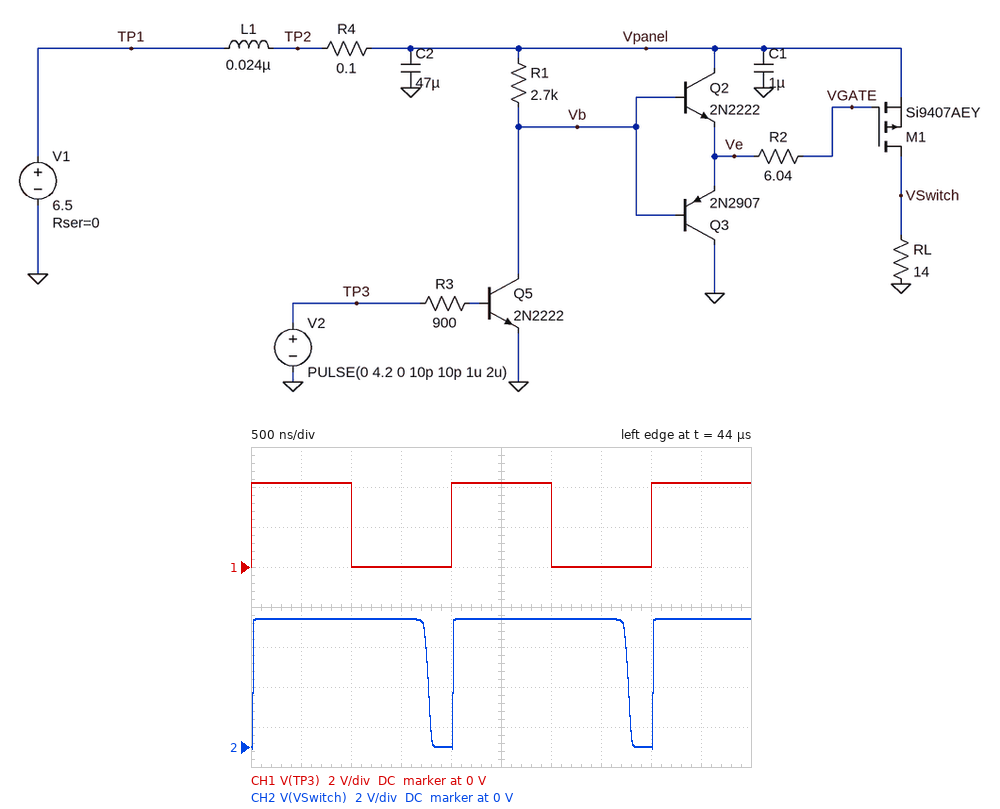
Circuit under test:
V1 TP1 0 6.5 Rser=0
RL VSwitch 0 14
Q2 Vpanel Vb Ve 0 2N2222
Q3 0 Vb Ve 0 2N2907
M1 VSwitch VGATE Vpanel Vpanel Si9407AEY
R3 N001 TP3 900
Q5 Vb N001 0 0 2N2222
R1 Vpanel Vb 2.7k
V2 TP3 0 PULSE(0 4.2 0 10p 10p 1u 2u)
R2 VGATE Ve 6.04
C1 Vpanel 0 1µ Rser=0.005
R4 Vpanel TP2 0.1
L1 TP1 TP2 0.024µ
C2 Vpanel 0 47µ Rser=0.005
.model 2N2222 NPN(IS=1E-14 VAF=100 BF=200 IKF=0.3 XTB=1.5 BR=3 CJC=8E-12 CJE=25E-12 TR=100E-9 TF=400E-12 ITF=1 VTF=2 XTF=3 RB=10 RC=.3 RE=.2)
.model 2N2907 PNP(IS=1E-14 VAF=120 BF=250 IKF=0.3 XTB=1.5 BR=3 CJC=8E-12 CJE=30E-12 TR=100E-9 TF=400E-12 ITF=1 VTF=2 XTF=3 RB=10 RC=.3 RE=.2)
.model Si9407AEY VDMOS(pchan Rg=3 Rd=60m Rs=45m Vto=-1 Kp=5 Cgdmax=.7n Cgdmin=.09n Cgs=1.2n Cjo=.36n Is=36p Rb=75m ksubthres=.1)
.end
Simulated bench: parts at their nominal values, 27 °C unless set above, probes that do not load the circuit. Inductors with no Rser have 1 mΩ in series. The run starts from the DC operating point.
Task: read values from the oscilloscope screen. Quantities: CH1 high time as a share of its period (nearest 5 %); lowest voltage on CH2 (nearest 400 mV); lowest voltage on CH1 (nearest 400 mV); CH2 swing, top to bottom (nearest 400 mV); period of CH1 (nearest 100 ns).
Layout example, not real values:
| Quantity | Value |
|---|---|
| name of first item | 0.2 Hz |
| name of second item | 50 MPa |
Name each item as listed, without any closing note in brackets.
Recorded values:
| Quantity | Value |
|---|---|
| CH1 high time as a share of its period | 50 % |
| lowest voltage on CH2 | 0 V |
| lowest voltage on CH1 | 0 V |
| CH2 swing, top to bottom | 6.4 V |
| period of CH1 | 2.0 µs |
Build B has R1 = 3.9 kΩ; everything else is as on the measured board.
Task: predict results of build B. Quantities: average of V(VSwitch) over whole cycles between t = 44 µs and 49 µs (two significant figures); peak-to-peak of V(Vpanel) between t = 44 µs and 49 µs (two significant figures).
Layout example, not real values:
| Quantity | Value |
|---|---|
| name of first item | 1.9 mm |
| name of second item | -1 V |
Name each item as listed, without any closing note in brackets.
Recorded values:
| Quantity | Value |
|---|---|
| average of V(VSwitch) over whole cycles between t = 44 µs and 49 µs | 5.9 V |
| peak-to-peak of V(Vpanel) between t = 44 µs and 49 µs | 3.3 mV |
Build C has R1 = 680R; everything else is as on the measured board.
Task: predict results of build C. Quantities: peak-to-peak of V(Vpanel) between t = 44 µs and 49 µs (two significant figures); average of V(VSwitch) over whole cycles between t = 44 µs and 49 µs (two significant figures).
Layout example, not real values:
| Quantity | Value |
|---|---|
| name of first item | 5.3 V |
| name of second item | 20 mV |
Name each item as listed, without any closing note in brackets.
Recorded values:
| Quantity | Value |
|---|---|
| peak-to-peak of V(Vpanel) between t = 44 µs and 49 µs | 5.1 mV |
| average of V(VSwitch) over whole cycles between t = 44 µs and 49 µs | 5.1 V |
